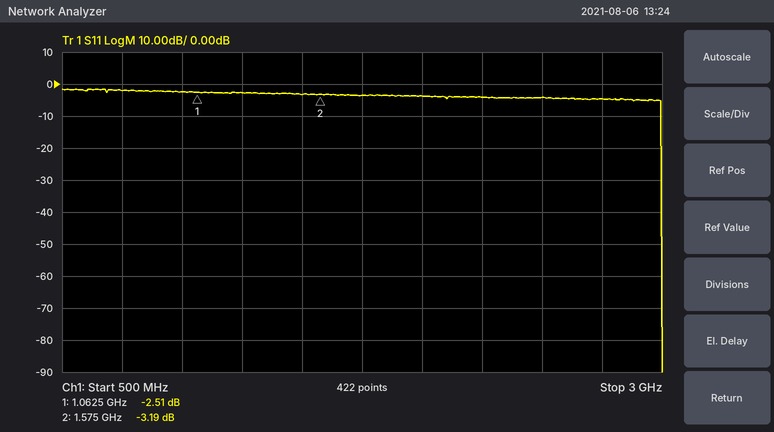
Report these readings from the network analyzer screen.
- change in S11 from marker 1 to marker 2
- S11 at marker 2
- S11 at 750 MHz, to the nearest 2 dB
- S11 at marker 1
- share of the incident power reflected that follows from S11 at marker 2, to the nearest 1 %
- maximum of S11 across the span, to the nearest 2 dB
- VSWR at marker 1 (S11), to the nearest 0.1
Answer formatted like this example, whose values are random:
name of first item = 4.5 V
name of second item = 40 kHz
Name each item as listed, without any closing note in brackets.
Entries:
change in S11 from marker 1 to marker 2 = -0.68 dB
S11 at marker 2 = -3.19 dB
S11 at 750 MHz, to the nearest 2 dB = -2 dB
S11 at marker 1 = -2.51 dB
share of the incident power reflected that follows from S11 at marker 2, to the nearest 1 % = 48 %
maximum of S11 across the span, to the nearest 2 dB = -2 dB
VSWR at marker 1 (S11), to the nearest 0.1 = 7.0
